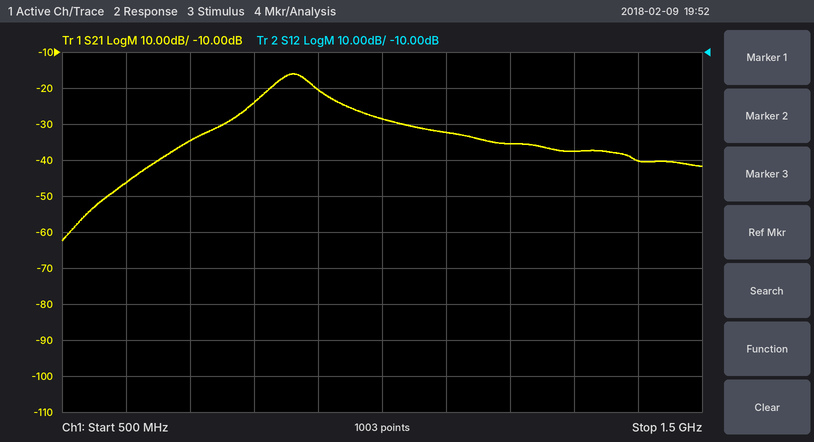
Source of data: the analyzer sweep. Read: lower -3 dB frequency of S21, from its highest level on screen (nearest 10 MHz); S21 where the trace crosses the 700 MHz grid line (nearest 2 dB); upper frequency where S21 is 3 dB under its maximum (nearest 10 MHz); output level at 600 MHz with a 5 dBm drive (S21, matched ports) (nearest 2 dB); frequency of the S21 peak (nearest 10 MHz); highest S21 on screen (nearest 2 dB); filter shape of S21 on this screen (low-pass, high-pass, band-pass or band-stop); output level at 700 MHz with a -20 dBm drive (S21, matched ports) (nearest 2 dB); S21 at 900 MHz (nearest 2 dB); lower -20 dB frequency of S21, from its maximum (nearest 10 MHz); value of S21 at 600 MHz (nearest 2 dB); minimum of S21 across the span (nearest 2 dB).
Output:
830 MHz
-34 dB
890 MHz
-42 dBm
860 MHz
-16 dB
band-pass
-54 dBm
-20 dB
690 MHz
-46 dB
-62 dB
